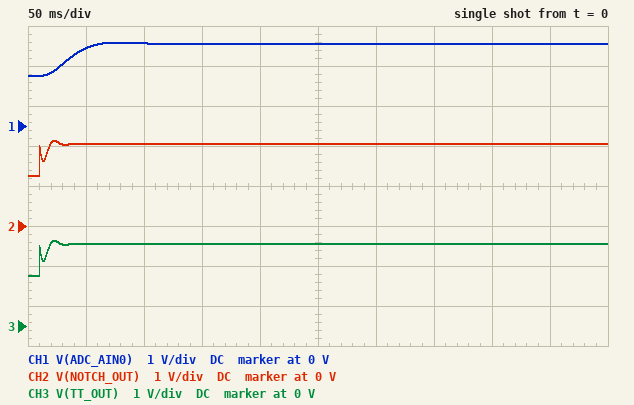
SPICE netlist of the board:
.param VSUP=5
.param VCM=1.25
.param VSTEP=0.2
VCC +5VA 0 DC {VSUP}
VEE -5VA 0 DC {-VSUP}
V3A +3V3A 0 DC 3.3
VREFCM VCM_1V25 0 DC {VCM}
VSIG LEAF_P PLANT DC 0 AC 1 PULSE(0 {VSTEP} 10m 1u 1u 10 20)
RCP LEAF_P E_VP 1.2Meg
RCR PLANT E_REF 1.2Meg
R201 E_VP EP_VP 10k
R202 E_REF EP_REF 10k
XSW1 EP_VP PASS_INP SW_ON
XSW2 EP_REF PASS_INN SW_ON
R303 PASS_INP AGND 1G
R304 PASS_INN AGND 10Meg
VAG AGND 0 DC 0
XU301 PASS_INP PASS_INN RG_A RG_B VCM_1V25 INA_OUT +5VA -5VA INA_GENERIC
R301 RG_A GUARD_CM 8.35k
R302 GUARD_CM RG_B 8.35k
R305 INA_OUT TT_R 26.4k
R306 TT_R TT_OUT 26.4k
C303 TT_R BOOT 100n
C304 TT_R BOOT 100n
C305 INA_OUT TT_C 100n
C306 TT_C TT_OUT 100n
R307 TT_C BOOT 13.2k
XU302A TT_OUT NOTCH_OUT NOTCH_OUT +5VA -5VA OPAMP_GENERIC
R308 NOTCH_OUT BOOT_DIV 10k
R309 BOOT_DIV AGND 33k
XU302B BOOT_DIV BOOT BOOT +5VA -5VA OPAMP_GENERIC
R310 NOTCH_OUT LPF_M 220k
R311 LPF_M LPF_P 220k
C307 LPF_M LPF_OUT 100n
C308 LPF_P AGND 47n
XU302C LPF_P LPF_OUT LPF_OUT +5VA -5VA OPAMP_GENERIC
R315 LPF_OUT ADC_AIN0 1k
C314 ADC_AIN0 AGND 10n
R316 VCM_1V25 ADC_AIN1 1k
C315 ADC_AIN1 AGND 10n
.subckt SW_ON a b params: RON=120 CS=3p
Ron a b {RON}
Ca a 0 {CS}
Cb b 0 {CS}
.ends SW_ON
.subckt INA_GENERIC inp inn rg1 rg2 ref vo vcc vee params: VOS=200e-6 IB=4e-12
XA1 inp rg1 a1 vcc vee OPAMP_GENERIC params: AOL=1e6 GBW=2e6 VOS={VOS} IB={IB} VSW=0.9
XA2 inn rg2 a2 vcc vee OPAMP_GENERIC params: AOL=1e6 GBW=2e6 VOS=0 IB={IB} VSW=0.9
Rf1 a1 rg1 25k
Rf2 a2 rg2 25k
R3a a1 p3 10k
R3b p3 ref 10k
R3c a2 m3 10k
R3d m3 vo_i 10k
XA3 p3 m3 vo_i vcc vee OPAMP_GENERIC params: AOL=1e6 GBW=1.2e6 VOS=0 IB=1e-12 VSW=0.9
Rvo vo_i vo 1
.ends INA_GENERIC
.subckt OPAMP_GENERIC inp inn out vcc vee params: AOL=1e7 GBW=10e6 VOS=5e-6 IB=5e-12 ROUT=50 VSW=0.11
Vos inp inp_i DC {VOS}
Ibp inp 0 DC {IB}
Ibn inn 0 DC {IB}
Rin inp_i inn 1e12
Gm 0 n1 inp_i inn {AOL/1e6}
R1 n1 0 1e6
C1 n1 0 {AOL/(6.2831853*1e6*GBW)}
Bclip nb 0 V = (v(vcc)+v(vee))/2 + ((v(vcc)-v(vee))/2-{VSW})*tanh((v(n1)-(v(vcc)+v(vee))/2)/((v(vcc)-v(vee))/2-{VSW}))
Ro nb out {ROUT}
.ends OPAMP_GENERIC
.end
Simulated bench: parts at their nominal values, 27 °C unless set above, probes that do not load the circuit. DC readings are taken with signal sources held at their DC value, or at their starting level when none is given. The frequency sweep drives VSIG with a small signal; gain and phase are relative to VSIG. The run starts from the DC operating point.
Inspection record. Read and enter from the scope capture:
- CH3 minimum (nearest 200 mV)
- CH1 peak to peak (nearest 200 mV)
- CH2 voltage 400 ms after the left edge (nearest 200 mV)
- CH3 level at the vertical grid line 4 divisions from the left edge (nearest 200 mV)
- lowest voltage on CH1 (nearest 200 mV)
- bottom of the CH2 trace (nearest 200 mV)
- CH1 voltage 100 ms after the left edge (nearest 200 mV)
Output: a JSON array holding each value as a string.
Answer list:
["1.2 V", "800 mV", "2.0 V", "2.0 V", "1.2 V", "1.2 V", "2.0 V"]
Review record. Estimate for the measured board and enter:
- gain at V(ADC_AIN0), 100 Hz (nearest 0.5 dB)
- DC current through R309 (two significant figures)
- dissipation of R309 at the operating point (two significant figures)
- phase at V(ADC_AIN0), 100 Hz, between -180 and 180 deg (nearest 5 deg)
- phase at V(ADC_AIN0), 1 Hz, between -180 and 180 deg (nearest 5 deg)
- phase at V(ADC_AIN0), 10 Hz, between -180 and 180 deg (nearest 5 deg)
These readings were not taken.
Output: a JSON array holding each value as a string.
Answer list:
["-29.5 dB", "29 µA", "28 µW", "-130 deg", "-10 deg", "-95 deg"]
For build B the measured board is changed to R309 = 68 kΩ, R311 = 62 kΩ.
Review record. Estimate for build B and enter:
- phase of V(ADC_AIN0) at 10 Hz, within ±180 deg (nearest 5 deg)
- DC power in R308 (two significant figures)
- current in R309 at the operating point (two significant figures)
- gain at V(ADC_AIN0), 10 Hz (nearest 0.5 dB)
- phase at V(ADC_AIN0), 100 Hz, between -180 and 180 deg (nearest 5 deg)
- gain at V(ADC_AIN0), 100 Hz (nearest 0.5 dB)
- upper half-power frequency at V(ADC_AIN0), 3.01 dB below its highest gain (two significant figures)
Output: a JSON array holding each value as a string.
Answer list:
["-55 deg", "2.6 µW", "16 µA", "11.0 dB", "-135 deg", "-17.0 dB", "16 Hz"]
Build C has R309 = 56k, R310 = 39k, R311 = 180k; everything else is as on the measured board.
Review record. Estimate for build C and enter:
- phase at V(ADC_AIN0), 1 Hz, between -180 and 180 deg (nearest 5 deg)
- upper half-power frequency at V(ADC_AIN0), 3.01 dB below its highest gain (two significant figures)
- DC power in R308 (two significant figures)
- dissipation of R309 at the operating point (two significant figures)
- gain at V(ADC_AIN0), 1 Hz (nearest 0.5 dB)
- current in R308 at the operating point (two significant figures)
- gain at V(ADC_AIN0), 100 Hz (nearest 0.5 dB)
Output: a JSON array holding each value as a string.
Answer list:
["-5 deg", "20 Hz", "3.6 µW", "20 µW", "12.0 dB", "19 µA", "-12.0 dB"]
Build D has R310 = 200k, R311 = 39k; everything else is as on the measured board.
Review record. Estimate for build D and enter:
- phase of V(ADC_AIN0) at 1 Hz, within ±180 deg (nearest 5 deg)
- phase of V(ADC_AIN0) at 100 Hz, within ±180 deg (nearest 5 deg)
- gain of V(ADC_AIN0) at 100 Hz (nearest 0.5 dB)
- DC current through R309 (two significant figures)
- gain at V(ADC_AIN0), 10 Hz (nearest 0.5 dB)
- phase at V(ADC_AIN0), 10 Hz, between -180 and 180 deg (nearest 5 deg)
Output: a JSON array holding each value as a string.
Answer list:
["-5 deg", "-110 deg", "-14.0 dB", "29 µA", "11.0 dB", "-50 deg"]
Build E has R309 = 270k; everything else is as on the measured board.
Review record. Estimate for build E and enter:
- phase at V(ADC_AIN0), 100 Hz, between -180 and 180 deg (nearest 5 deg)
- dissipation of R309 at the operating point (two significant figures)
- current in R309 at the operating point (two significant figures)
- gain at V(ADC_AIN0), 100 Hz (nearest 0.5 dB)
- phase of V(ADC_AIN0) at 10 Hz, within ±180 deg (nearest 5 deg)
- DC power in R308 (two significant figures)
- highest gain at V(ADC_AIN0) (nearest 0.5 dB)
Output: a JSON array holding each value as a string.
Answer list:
["-165 deg", "5.4 µW", "4.5 µA", "-27.0 dB", "-85 deg", "200 nW", "12.0 dB"]
